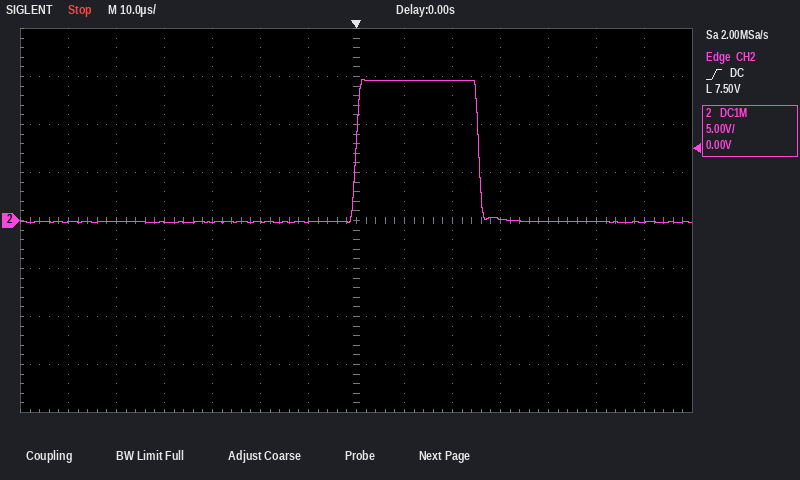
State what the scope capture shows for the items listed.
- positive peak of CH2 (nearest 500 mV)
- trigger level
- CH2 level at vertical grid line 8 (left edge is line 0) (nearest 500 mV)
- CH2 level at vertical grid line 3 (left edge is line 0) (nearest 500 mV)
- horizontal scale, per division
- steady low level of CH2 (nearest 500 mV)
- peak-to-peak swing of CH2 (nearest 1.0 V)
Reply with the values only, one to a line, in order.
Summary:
14.5 V
7.50 V
14.5 V
0.0 V
10 µs
0.0 V
15.0 V
